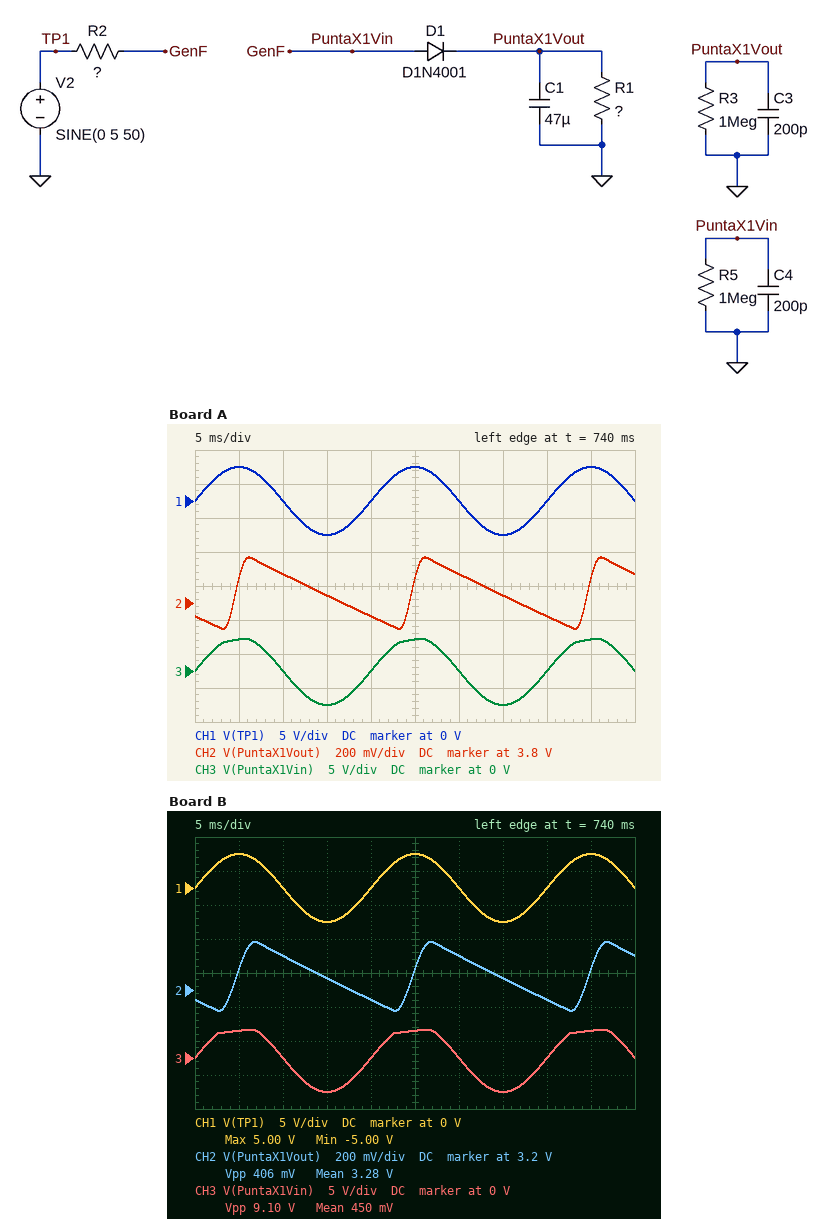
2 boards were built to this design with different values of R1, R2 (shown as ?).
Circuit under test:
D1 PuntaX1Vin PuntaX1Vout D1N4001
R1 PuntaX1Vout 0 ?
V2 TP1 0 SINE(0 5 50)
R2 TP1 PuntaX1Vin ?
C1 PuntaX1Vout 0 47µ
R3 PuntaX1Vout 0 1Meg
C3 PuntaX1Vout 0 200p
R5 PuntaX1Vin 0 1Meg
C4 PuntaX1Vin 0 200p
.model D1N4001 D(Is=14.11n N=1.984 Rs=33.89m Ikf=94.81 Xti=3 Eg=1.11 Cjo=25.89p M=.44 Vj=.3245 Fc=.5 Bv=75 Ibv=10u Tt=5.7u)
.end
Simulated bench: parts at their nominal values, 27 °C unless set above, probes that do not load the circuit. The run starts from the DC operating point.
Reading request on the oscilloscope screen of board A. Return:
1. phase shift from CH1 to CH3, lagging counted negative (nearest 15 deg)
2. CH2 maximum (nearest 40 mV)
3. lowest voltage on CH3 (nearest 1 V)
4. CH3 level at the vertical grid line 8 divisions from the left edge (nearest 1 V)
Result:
0 deg
4.08 V
-5 V
0 V
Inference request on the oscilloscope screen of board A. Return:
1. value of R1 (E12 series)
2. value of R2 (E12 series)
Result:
3.3 kΩ
33 Ω
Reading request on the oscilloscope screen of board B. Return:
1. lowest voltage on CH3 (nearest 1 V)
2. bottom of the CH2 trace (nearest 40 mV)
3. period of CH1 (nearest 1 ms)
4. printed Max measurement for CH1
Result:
-5 V
3.08 V
20 ms
5.00 V
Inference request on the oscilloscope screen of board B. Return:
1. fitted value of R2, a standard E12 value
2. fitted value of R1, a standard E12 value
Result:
120 Ω
2.7 kΩ
